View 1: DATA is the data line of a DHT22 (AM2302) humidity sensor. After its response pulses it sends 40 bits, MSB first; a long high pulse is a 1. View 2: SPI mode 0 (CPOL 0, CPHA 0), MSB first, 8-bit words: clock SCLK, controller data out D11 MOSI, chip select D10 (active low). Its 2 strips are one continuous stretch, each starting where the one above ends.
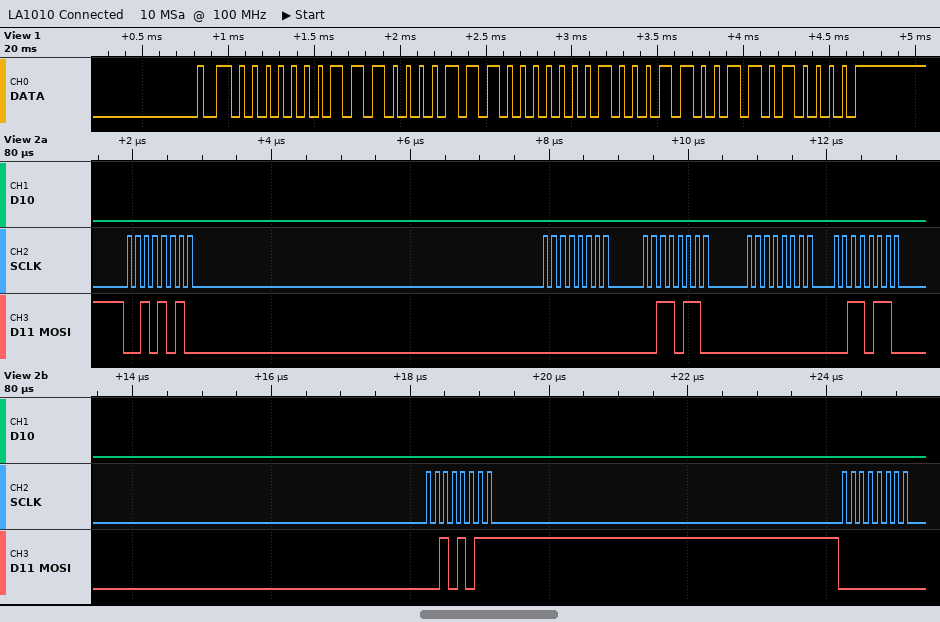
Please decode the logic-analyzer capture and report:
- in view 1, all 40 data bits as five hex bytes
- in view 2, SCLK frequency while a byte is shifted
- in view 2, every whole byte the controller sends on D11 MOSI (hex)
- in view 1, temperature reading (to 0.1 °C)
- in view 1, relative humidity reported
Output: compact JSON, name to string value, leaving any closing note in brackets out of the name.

{"in view 1, all 40 data bits as five hex bytes": "01 C3 80 8C D0", "in view 2, SCLK frequency while a byte is shifted": "8 MHz", "in view 2, every whole byte the controller sends on D11 MOSI": "2A 00 36 00 36 2B 00", "in view 1, temperature reading": "-14.0 °C", "in view 1, relative humidity reported": "45.1 %"}
